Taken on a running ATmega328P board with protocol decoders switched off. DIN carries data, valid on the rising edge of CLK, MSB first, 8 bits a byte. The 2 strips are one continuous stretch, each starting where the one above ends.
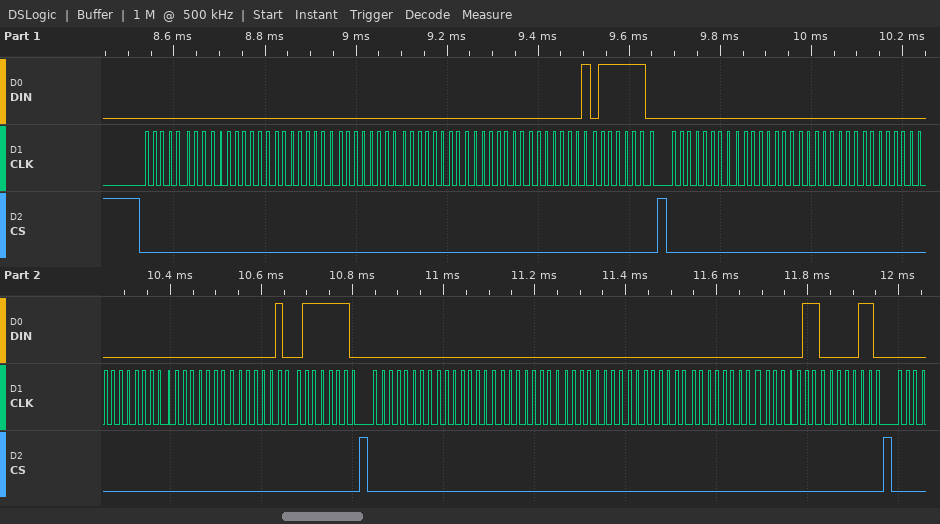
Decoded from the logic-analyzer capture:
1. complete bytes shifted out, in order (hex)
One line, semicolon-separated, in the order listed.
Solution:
0x00 0x00 0x00 0x00 0x00 0x00 0x01 0x7E 0x00 0x00 0x00 0x00 0x00 0x00 0x02 0x7E 0x00 0x00 0x00 0x00 0x00 0x00 0x03 0x06
